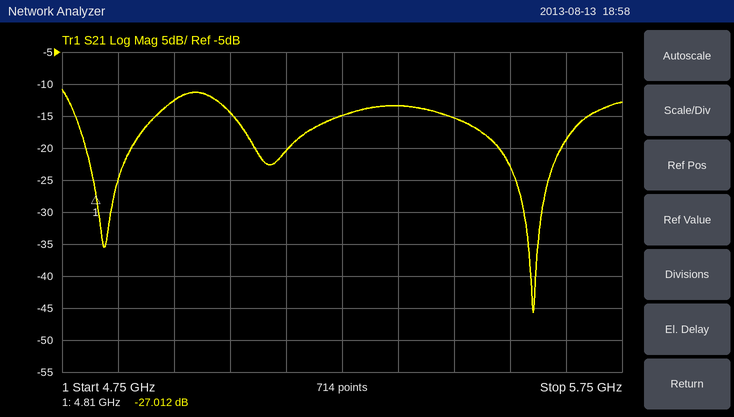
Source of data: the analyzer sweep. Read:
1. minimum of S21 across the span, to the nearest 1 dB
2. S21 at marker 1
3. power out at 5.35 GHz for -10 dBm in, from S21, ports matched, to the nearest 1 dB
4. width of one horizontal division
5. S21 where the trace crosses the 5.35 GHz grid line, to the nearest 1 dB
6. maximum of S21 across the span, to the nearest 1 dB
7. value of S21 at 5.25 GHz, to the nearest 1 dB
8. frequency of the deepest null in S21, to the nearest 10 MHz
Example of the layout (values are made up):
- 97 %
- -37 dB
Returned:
- -46 dB
- -27.012 dB
- -23 dBm
- 100 MHz
- -13 dB
- -11 dB
- -15 dB
- 5.59 GHz
